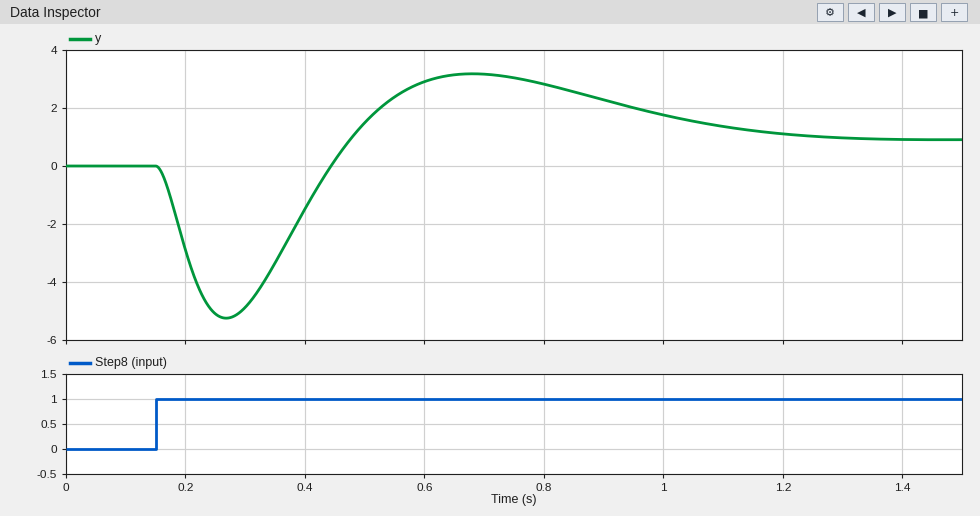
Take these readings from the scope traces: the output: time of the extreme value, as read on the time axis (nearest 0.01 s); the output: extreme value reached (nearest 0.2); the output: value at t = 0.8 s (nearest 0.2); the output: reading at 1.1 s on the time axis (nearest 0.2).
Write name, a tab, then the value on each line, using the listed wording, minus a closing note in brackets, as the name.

the output: time of the extreme value, as read on the time axis	0.27 s
the output: extreme value reached	-5.2
the output: value at t = 0.8 s	2.8
the output: reading at 1.1 s on the time axis	1.4
